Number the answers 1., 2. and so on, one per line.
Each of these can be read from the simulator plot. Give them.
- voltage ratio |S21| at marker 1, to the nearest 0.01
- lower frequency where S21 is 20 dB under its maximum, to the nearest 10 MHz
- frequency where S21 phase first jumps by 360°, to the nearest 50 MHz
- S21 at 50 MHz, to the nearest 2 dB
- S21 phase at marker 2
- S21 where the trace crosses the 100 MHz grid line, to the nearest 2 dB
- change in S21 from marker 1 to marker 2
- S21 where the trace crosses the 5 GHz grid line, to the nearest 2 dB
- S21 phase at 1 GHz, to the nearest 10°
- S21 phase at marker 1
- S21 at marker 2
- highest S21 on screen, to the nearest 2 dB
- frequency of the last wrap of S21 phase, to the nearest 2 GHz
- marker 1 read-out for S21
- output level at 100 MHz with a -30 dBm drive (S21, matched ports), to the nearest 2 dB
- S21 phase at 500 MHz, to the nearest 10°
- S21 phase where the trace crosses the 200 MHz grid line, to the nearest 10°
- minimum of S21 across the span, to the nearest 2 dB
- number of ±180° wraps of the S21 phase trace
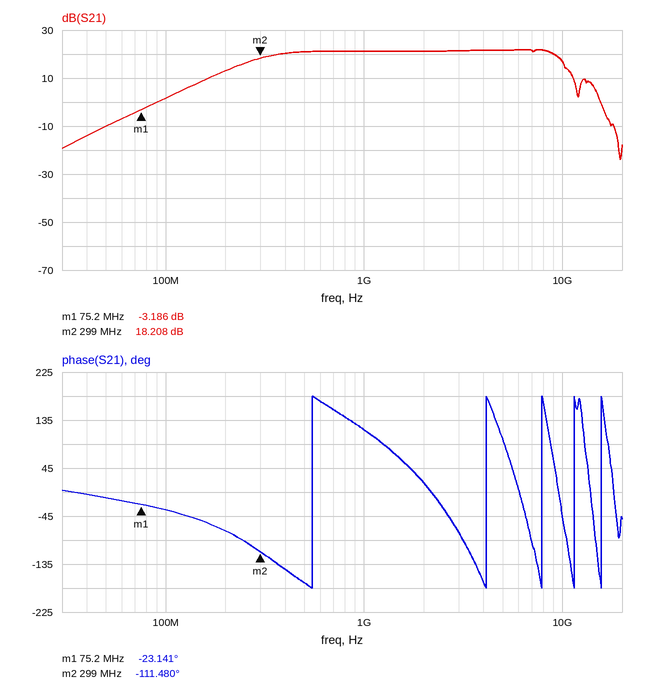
1. 0.69
2. 100 MHz
3. 550 MHz
4. -10 dB
5. -111.480°
6. 2 dB
7. 21.394 dB
8. 22 dB
9. 120°
10. -23.141°
11. 18.208 dB
12. 22 dB
13. 16 GHz
14. -3.186 dB
15. -28 dBm
16. -170°
17. -70°
18. -24 dB
19. 5
